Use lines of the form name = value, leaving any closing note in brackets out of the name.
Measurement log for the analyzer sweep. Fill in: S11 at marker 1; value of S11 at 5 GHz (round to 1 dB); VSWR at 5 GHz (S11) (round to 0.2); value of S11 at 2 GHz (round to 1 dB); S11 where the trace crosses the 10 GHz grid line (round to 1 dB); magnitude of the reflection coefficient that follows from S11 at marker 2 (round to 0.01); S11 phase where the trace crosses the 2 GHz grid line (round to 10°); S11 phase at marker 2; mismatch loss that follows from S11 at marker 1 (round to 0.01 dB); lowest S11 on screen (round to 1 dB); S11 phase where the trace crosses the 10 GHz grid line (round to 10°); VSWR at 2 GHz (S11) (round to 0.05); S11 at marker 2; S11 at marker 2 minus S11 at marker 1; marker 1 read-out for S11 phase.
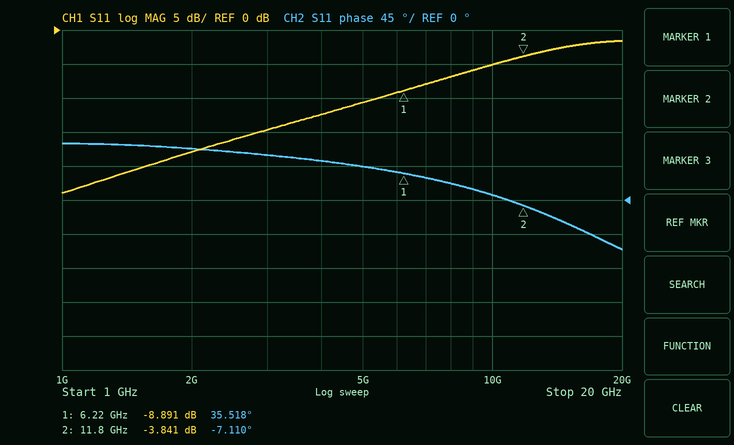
S11 at marker 1 = -8.891 dB
value of S11 at 5 GHz = -11 dB
VSWR at 5 GHz (S11) = 1.8
value of S11 at 2 GHz = -18 dB
S11 where the trace crosses the 10 GHz grid line = -5 dB
magnitude of the reflection coefficient that follows from S11 at marker 2 = 0.64
S11 phase where the trace crosses the 2 GHz grid line = 70°
S11 phase at marker 2 = -7.110°
mismatch loss that follows from S11 at marker 1 = 0.60 dB
lowest S11 on screen = -24 dB
S11 phase where the trace crosses the 10 GHz grid line = 10°
VSWR at 2 GHz (S11) = 1.30
S11 at marker 2 = -3.841 dB
S11 at marker 2 minus S11 at marker 1 = 5.050 dB
marker 1 read-out for S11 phase = 35.518°
